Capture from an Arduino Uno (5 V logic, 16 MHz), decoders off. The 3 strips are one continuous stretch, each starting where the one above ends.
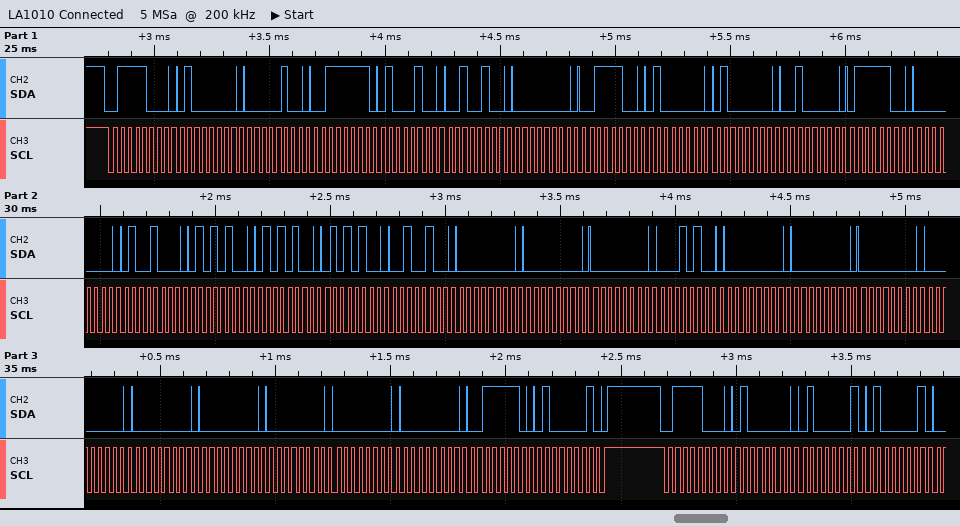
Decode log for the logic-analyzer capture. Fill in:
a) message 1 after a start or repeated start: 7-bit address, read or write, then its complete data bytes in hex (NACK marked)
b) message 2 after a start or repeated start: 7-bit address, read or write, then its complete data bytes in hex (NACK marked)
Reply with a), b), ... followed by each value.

a) 0x3C write: 40 04 3F 44 24 00 3C 40 40 20 7C 00 48 54 54 54 24 00 00 00 14 00 00 00 00 00 00 00 00 00 3E 41
b) 0x3C write: 40 41 41
